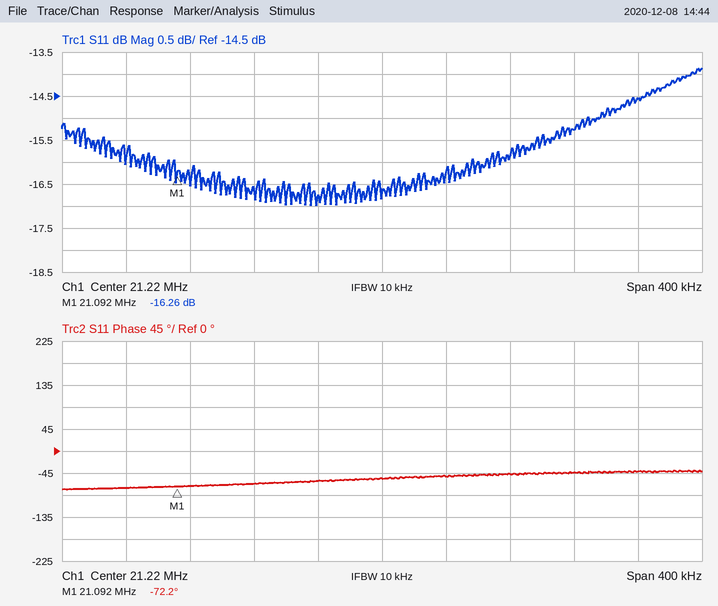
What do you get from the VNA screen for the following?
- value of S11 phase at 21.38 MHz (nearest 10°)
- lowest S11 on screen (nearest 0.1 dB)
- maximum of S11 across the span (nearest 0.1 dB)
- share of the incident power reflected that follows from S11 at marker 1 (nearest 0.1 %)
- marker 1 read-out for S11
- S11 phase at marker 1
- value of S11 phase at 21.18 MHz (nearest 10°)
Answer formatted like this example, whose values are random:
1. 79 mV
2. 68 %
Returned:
1. -40°
2. -17.0 dB
3. -13.9 dB
4. 2.4 %
5. -16.26 dB
6. -72.2°
7. -60°
